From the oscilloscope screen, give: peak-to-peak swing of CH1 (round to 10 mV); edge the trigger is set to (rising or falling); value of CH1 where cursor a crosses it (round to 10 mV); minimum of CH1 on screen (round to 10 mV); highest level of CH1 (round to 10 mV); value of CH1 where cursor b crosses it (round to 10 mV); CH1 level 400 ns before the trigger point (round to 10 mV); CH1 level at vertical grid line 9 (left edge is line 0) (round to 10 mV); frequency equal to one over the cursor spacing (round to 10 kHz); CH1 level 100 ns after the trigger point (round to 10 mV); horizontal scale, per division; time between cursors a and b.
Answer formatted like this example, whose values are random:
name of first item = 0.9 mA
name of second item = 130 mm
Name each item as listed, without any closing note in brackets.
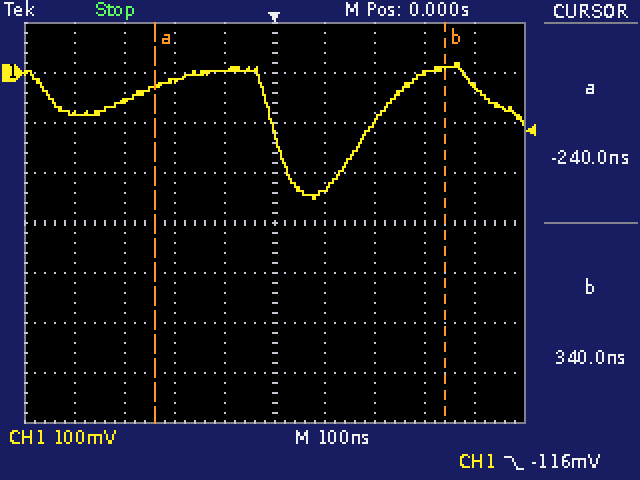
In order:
peak-to-peak swing of CH1 = 270 mV
edge the trigger is set to = falling
value of CH1 where cursor a crosses it = -30 mV
minimum of CH1 on screen = -250 mV
highest level of CH1 = 20 mV
value of CH1 where cursor b crosses it = 10 mV
CH1 level 400 ns before the trigger point = -80 mV
CH1 level at vertical grid line 9 (left edge is line 0) = -30 mV
frequency equal to one over the cursor spacing = 1.72 MHz
CH1 level 100 ns after the trigger point = -230 mV
horizontal scale, per division = 100 ns
time between cursors a and b = 580 ns
